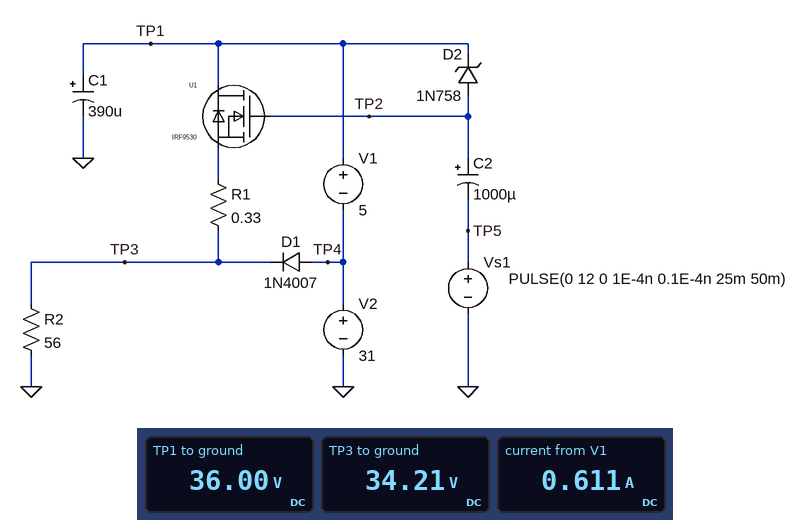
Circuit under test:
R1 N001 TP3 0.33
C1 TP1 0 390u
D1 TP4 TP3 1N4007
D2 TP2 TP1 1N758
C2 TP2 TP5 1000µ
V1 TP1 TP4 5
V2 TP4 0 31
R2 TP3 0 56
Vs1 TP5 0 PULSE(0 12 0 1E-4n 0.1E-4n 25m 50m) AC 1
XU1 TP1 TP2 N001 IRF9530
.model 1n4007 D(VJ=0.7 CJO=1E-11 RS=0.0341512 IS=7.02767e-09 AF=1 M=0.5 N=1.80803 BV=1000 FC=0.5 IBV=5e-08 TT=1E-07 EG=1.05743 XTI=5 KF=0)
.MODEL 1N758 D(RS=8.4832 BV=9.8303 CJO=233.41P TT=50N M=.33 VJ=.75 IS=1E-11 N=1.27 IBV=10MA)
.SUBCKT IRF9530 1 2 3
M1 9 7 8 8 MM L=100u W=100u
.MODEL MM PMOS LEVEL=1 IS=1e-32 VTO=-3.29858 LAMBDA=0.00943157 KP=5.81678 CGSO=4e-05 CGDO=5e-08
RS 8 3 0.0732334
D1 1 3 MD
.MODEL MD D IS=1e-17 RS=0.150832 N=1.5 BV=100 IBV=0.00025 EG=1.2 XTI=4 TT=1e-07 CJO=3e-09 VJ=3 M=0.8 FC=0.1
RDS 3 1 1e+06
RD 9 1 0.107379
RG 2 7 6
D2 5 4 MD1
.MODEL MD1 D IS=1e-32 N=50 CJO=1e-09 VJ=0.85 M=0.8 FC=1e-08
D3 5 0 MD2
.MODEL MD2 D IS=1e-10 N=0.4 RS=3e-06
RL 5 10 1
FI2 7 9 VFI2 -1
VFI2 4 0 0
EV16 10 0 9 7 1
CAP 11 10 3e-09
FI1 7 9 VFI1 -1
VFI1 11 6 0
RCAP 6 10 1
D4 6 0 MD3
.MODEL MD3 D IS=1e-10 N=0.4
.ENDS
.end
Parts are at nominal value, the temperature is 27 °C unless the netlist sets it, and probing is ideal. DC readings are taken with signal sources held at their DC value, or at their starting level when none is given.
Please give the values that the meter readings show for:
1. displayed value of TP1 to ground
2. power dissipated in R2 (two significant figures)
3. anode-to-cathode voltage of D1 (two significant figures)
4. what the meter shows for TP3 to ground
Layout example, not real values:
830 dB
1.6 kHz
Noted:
36.00 V
21 W
-3.2 V
34.21 V
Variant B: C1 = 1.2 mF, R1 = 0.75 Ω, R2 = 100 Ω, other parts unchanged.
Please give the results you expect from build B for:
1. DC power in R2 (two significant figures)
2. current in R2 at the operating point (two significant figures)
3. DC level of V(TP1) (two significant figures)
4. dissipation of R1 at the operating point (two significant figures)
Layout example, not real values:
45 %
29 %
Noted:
12 W
340 mA
36 V
88 mW
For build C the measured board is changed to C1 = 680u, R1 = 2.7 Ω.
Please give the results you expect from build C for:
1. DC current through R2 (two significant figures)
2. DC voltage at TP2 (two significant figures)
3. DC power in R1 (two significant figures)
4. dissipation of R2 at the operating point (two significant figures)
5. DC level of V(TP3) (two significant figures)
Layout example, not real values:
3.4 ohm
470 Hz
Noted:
590 mA
36 V
930 mW
19 W
33 V
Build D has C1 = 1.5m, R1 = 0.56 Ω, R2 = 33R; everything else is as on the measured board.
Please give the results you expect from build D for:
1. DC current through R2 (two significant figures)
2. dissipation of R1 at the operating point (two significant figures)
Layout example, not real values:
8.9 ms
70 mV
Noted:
1.0 A
590 mW
